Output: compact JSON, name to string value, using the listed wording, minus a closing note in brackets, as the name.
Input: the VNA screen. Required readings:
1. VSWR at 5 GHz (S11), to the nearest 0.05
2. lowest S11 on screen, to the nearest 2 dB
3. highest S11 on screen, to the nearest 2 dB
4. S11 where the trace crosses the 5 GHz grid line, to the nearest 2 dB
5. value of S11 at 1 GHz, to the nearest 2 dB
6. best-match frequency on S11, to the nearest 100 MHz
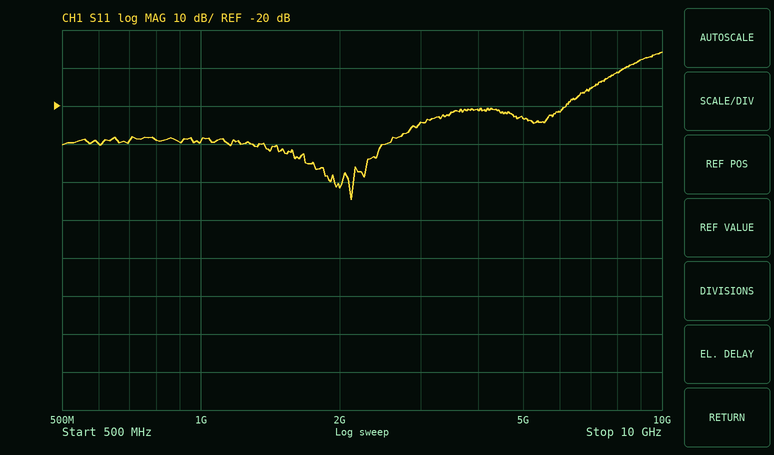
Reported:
{"VSWR at 5 GHz (S11), to the nearest 0.05": "1.15", "lowest S11 on screen, to the nearest 2 dB": "-44 dB", "highest S11 on screen, to the nearest 2 dB": "-6 dB", "S11 where the trace crosses the 5 GHz grid line, to the nearest 2 dB": "-24 dB", "value of S11 at 1 GHz, to the nearest 2 dB": "-30 dB", "best-match frequency on S11, to the nearest 100 MHz": "2.1 GHz"}
